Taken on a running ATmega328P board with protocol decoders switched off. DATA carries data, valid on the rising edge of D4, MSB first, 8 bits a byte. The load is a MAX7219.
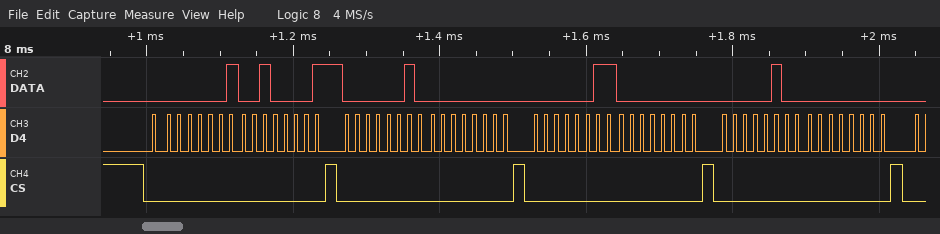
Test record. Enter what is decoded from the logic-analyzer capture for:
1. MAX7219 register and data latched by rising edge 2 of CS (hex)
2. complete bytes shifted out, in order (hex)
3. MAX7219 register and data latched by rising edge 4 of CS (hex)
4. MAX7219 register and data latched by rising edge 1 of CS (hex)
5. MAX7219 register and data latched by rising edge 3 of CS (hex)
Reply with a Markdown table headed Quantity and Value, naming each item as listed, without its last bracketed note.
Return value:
| Quantity | Value |
|---|---|
| MAX7219 register and data latched by rising edge 2 of CS | register 0x2, data 0x00 |
| complete bytes shifted out, in order | 01 21 02 00 03 00 04 00 |
| MAX7219 register and data latched by rising edge 4 of CS | register 0x4, data 0x00 |
| MAX7219 register and data latched by rising edge 1 of CS | register 0x1, data 0x21 |
| MAX7219 register and data latched by rising edge 3 of CS | register 0x3, data 0x00 |
